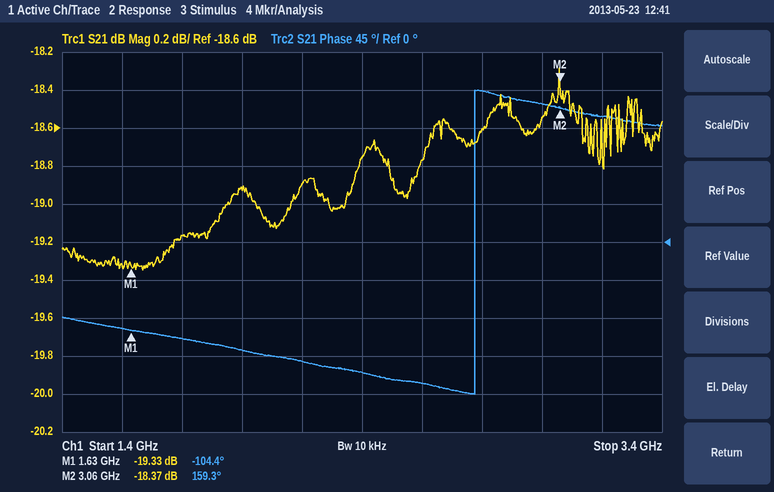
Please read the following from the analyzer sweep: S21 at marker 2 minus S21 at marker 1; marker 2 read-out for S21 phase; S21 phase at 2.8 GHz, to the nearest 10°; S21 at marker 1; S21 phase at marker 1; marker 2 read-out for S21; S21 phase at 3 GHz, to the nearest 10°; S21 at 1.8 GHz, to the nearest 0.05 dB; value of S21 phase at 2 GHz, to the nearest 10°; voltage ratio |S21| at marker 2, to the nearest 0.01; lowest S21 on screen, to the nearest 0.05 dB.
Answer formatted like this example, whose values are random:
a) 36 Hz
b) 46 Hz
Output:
a) 0.96 dB
b) 159.3°
c) 180°
d) -19.33 dB
e) -104.4°
f) -18.37 dB
g) 160°
h) -19.15 dB
i) -130°
j) 0.12
k) -19.35 dB
